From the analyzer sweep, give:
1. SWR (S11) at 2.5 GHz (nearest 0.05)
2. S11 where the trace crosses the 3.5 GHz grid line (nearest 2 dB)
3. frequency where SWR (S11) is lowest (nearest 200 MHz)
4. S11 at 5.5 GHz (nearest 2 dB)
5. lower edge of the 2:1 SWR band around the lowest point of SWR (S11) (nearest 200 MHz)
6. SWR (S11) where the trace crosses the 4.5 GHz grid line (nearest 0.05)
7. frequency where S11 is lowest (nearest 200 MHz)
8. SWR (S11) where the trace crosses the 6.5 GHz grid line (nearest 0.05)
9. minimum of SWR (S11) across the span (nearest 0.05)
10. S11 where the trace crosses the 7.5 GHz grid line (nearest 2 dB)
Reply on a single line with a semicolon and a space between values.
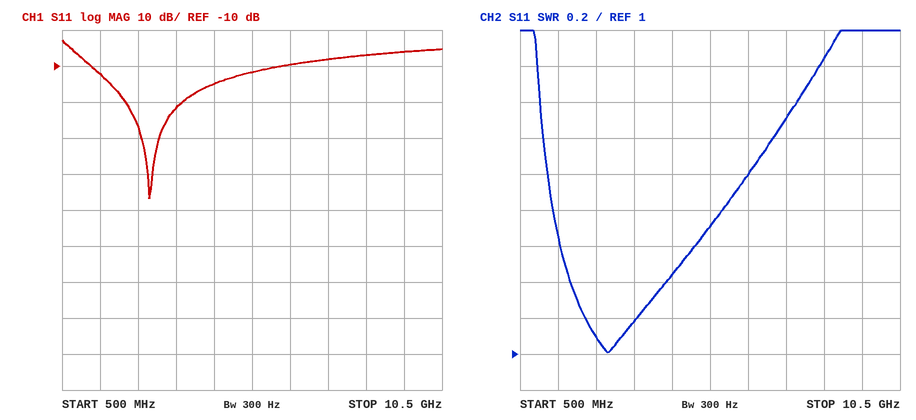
1.10; -22 dB; 2.8 GHz; -12 dB; 1.2 GHz; 1.45; 2.8 GHz; 2.00; 1.00; -8 dB
